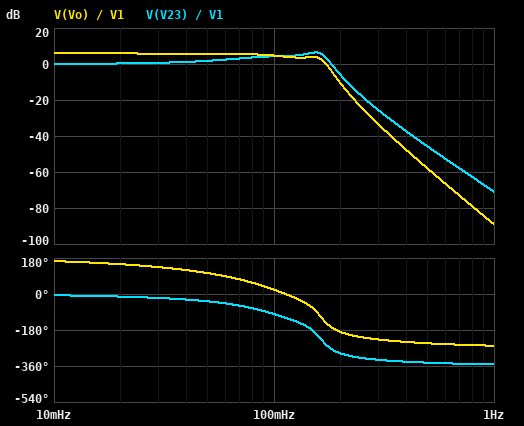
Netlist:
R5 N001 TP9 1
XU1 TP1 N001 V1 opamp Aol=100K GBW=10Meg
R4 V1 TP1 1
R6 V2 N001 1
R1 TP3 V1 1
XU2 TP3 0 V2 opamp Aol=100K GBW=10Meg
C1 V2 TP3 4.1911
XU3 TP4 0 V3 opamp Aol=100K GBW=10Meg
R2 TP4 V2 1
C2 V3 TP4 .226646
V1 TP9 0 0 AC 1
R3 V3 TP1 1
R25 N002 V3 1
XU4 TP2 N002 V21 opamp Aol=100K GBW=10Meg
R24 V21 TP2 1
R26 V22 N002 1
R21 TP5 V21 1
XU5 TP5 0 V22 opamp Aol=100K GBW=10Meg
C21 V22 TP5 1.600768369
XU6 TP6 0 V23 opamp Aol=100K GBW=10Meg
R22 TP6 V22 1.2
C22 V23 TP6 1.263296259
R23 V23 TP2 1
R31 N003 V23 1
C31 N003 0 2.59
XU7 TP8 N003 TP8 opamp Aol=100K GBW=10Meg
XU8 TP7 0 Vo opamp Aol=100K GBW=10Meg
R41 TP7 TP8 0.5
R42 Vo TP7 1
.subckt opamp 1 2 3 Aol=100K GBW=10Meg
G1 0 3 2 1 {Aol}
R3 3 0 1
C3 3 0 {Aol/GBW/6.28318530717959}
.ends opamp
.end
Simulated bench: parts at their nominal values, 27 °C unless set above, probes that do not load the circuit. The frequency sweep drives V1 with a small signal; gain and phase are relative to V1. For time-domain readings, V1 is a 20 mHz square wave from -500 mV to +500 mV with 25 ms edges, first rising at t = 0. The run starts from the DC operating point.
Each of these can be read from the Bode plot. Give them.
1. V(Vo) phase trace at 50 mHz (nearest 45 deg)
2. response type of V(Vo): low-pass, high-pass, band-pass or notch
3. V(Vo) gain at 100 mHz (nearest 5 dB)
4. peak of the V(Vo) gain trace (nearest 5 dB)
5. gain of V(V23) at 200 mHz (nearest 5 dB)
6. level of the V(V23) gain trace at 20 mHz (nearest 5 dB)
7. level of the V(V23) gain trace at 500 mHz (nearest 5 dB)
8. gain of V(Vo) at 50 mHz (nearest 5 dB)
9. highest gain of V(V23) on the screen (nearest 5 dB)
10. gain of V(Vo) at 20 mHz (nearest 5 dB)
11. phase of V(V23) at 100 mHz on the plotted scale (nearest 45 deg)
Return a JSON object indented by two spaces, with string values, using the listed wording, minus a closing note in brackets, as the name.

{
  "V(Vo) phase trace at 50 mHz": "90 deg",
  "response type of V(Vo): low-pass, high-pass, band-pass or notch": "low-pass",
  "V(Vo) gain at 100 mHz": "5 dB",
  "peak of the V(Vo) gain trace": "5 dB",
  "gain of V(V23) at 200 mHz": "-5 dB",
  "level of the V(V23) gain trace at 20 mHz": "0 dB",
  "level of the V(V23) gain trace at 500 mHz": "-45 dB",
  "gain of V(Vo) at 50 mHz": "5 dB",
  "highest gain of V(V23) on the screen": "5 dB",
  "gain of V(Vo) at 20 mHz": "5 dB",
  "phase of V(V23) at 100 mHz on the plotted scale": "-90 deg"
}
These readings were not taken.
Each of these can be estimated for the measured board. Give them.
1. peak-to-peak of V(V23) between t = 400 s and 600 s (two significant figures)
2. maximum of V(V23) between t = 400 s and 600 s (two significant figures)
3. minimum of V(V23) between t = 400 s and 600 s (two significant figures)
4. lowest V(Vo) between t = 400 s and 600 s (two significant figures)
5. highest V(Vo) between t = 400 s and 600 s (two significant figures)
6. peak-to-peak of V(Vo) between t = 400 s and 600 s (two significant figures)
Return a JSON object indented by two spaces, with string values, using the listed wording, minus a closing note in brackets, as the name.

{
  "peak-to-peak of V(V23) between t = 400 s and 600 s": "2.0 V",
  "maximum of V(V23) between t = 400 s and 600 s": "1.0 V",
  "minimum of V(V23) between t = 400 s and 600 s": "-1.0 V",
  "lowest V(Vo) between t = 400 s and 600 s": "-1.2 V",
  "highest V(Vo) between t = 400 s and 600 s": "1.2 V",
  "peak-to-peak of V(Vo) between t = 400 s and 600 s": "2.3 V"
}
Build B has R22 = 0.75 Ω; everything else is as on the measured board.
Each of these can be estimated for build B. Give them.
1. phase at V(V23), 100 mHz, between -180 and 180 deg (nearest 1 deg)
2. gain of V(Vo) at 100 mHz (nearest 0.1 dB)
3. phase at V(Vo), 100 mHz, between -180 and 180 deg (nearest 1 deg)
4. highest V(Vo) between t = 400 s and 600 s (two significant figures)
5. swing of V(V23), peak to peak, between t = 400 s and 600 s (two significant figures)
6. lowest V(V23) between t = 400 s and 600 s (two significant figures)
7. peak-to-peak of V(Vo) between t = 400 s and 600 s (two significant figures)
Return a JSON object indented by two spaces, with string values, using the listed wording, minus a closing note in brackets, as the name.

{
  "phase at V(V23), 100 mHz, between -180 and 180 deg": "-69 deg",
  "gain of V(Vo) at 100 mHz": "7.1 dB",
  "phase at V(Vo), 100 mHz, between -180 and 180 deg": "53 deg",
  "highest V(Vo) between t = 400 s and 600 s": "1.4 V",
  "swing of V(V23), peak to peak, between t = 400 s and 600 s": "2.6 V",
  "lowest V(V23) between t = 400 s and 600 s": "-1.3 V",
  "peak-to-peak of V(Vo) between t = 400 s and 600 s": "2.8 V"
}
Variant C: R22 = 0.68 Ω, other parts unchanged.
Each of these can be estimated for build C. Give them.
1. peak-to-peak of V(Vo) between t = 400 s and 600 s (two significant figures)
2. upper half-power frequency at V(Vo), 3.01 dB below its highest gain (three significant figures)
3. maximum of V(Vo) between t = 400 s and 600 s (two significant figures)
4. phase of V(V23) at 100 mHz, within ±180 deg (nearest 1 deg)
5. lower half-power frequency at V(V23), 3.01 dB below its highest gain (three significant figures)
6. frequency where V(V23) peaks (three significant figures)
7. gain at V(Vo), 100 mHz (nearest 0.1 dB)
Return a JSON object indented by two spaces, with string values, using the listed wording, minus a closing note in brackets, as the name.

{
  "peak-to-peak of V(Vo) between t = 400 s and 600 s": "2.9 V",
  "upper half-power frequency at V(Vo), 3.01 dB below its highest gain": "170 mHz",
  "maximum of V(Vo) between t = 400 s and 600 s": "1.4 V",
  "phase of V(V23) at 100 mHz, within ±180 deg": "-63 deg",
  "lower half-power frequency at V(V23), 3.01 dB below its highest gain": "127 mHz",
  "frequency where V(V23) peaks": "156 mHz",
  "gain at V(Vo), 100 mHz": "7.3 dB"
}
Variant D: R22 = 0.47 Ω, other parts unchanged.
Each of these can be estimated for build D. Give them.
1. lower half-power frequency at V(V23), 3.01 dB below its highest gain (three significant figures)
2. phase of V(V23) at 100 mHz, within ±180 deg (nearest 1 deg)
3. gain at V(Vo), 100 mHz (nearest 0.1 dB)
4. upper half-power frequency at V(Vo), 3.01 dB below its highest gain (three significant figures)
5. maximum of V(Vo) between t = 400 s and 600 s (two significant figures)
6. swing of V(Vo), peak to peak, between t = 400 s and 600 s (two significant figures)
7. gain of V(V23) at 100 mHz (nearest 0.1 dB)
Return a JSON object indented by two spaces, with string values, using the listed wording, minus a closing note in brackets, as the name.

{
  "lower half-power frequency at V(V23), 3.01 dB below its highest gain": "140 mHz",
  "phase of V(V23) at 100 mHz, within ±180 deg": "-44 deg",
  "gain at V(Vo), 100 mHz": "7.0 dB",
  "upper half-power frequency at V(Vo), 3.01 dB below its highest gain": "173 mHz",
  "maximum of V(Vo) between t = 400 s and 600 s": "1.5 V",
  "swing of V(Vo), peak to peak, between t = 400 s and 600 s": "3.0 V",
  "gain of V(V23) at 100 mHz": "6.6 dB"
}
